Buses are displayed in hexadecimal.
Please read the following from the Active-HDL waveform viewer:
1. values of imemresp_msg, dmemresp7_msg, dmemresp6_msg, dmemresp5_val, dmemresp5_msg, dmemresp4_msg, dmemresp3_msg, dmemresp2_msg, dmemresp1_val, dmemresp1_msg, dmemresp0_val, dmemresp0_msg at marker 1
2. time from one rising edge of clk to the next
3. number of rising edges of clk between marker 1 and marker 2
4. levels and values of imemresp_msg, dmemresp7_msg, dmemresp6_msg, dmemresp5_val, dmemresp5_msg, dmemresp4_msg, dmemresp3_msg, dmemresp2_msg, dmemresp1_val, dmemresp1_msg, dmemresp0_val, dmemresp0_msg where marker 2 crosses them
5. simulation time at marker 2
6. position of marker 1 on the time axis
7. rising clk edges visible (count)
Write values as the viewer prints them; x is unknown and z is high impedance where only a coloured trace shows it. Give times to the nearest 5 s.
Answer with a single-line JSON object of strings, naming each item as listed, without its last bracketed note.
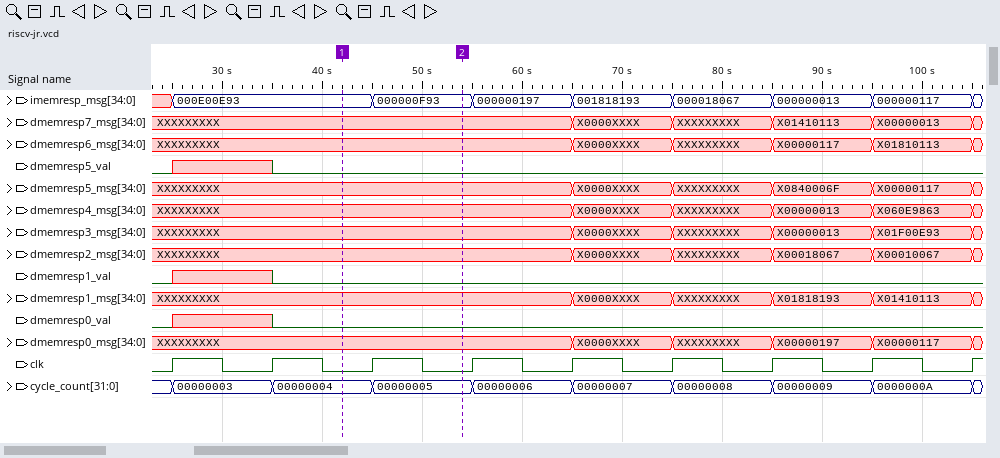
{"values of imemresp_msg, dmemresp7_msg, dmemresp6_msg, dmemresp5_val, dmemresp5_msg, dmemresp4_msg, dmemresp3_msg, dmemresp2_msg, dmemresp1_val, dmemresp1_msg, dmemresp0_val, dmemresp0_msg at marker 1": "imemresp_msg=000E00E93, dmemresp7_msg=XXXXXXXXX, dmemresp6_msg=XXXXXXXXX, dmemresp5_val=0, dmemresp5_msg=XXXXXXXXX, dmemresp4_msg=XXXXXXXXX, dmemresp3_msg=XXXXXXXXX, dmemresp2_msg=XXXXXXXXX, dmemresp1_val=0, dmemresp1_msg=XXXXXXXXX, dmemresp0_val=0, dmemresp0_msg=XXXXXXXXX", "time from one rising edge of clk to the next": "10 s", "number of rising edges of clk between marker 1 and marker 2": "1", "levels and values of imemresp_msg, dmemresp7_msg, dmemresp6_msg, dmemresp5_val, dmemresp5_msg, dmemresp4_msg, dmemresp3_msg, dmemresp2_msg, dmemresp1_val, dmemresp1_msg, dmemresp0_val, dmemresp0_msg where marker 2 crosses them": "imemresp_msg=000000F93, dmemresp7_msg=XXXXXXXXX, dmemresp6_msg=XXXXXXXXX, dmemresp5_val=0, dmemresp5_msg=XXXXXXXXX, dmemresp4_msg=XXXXXXXXX, dmemresp3_msg=XXXXXXXXX, dmemresp2_msg=XXXXXXXXX, dmemresp1_val=0, dmemresp1_msg=XXXXXXXXX, dmemresp0_val=0, dmemresp0_msg=XXXXXXXXX", "simulation time at marker 2": "55 s", "position of marker 1 on the time axis": "40 s", "rising clk edges visible": "9"}
